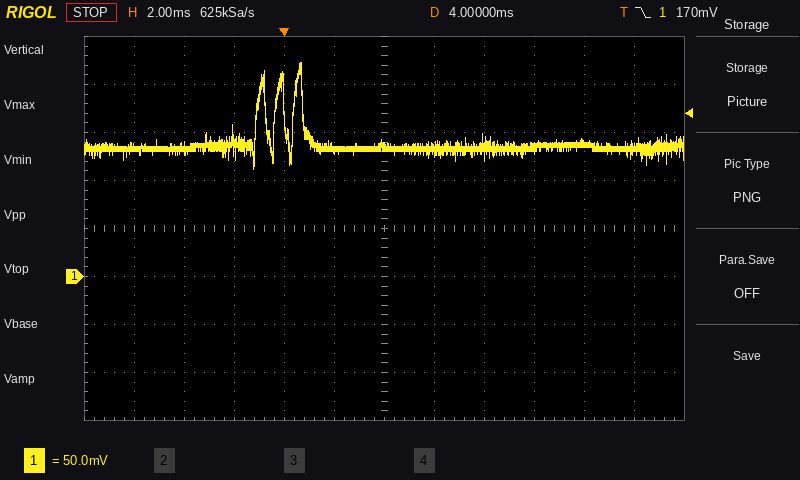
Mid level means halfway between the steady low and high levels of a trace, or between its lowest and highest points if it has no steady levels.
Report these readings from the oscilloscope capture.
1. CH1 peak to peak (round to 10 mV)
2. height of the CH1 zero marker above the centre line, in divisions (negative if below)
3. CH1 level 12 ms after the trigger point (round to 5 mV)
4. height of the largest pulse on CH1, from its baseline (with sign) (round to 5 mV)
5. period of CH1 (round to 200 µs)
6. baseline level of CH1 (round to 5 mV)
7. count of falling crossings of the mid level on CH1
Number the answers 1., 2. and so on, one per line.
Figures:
1. 110 mV
2. -1.0 div
3. 140 mV
4. +90 mV
5. 800 µs
6. 135 mV
7. 3
